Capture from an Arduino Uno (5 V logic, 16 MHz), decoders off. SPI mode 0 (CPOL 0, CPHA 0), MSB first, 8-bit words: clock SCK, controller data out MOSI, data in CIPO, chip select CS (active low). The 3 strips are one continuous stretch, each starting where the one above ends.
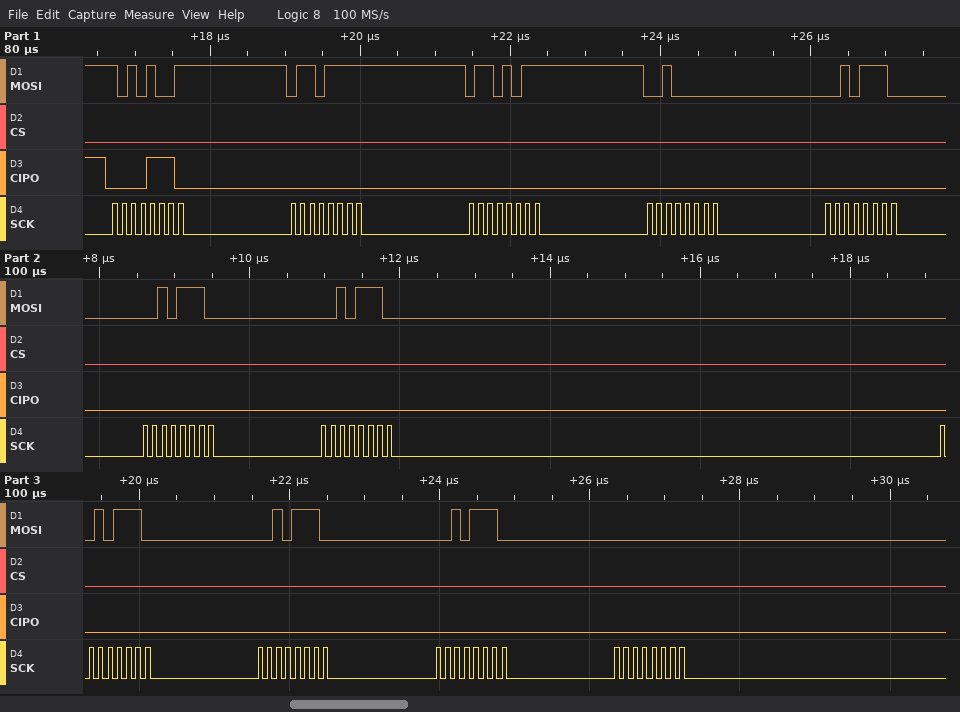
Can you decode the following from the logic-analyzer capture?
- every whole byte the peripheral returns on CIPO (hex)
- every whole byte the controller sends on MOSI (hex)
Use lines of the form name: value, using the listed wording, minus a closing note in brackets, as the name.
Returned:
every whole byte the peripheral returns on CIPO: 0x0E 0x00 0x00 0x00 0x00 0x00 0x00 0x00 0x00 0x00 0x00
every whole byte the controller sends on MOSI: 0xA9 0x6F 0x6B 0x20 0x2E 0x2E 0x2E 0x2E 0x2E 0x2E 0x00
